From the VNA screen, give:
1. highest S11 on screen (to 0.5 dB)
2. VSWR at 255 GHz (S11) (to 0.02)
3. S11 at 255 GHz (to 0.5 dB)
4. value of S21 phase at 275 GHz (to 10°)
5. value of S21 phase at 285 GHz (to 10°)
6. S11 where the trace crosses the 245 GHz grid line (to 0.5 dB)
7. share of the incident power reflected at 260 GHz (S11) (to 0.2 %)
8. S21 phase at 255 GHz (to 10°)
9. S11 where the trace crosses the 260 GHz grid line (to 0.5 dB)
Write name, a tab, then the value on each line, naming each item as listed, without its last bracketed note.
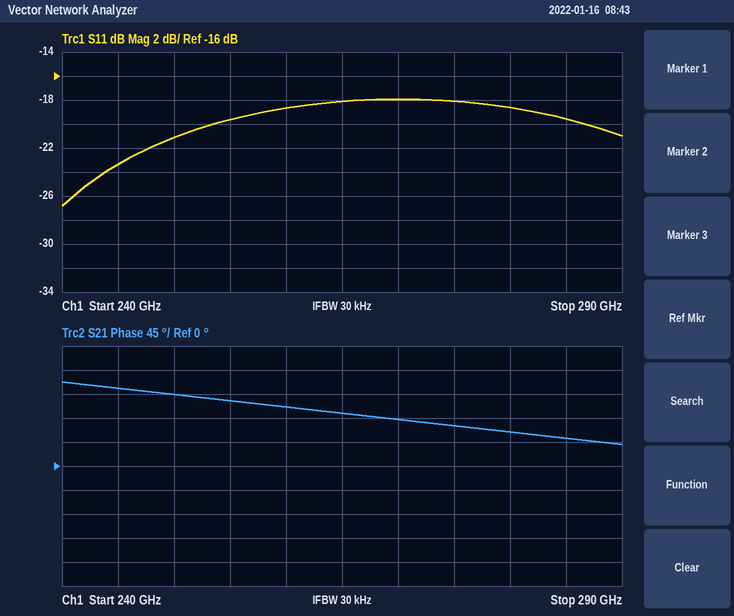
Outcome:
highest S11 on screen	-18.0 dB
VSWR at 255 GHz (S11)	1.24
S11 at 255 GHz	-19.5 dB
value of S21 phase at 275 GHz	80°
value of S21 phase at 285 GHz	50°
S11 where the trace crosses the 245 GHz grid line	-23.5 dB
share of the incident power reflected at 260 GHz (S11)	1.4 %
S21 phase at 255 GHz	120°
S11 where the trace crosses the 260 GHz grid line	-18.5 dB
